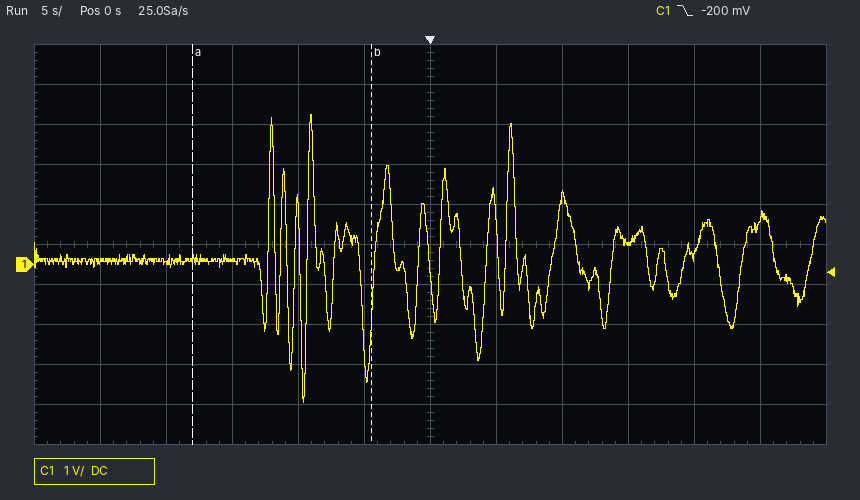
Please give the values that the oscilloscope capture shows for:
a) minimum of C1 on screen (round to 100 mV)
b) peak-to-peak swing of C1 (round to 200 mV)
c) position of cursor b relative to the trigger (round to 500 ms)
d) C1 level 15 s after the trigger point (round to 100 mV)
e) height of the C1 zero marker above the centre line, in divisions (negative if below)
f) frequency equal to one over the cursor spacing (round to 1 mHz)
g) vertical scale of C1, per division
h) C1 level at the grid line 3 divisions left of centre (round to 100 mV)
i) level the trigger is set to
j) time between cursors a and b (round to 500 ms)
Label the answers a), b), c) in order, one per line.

a) -3.4 V
b) 7.2 V
c) -4.5 s
d) 600 mV
e) -0.5 div
f) 74 mHz
g) 1 V
h) 100 mV
i) -200 mV
j) 13.5 s
